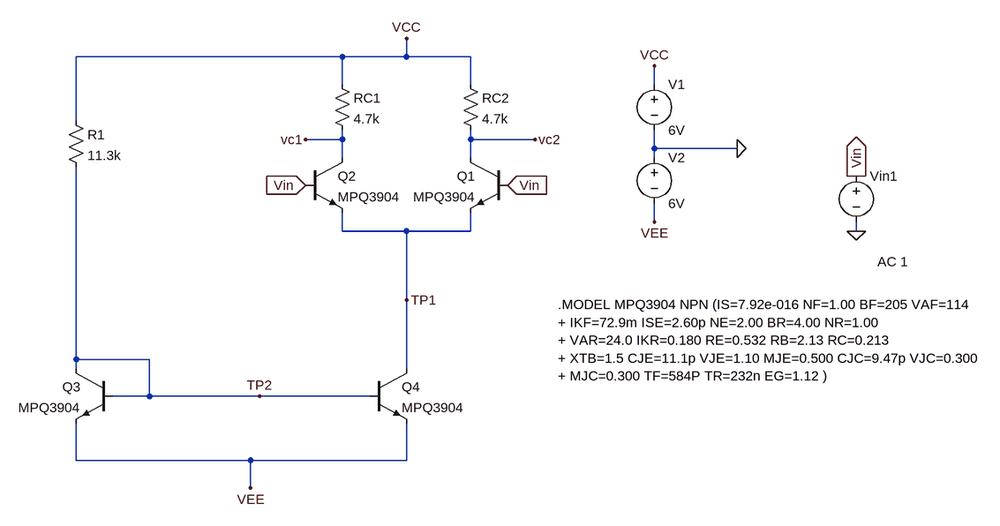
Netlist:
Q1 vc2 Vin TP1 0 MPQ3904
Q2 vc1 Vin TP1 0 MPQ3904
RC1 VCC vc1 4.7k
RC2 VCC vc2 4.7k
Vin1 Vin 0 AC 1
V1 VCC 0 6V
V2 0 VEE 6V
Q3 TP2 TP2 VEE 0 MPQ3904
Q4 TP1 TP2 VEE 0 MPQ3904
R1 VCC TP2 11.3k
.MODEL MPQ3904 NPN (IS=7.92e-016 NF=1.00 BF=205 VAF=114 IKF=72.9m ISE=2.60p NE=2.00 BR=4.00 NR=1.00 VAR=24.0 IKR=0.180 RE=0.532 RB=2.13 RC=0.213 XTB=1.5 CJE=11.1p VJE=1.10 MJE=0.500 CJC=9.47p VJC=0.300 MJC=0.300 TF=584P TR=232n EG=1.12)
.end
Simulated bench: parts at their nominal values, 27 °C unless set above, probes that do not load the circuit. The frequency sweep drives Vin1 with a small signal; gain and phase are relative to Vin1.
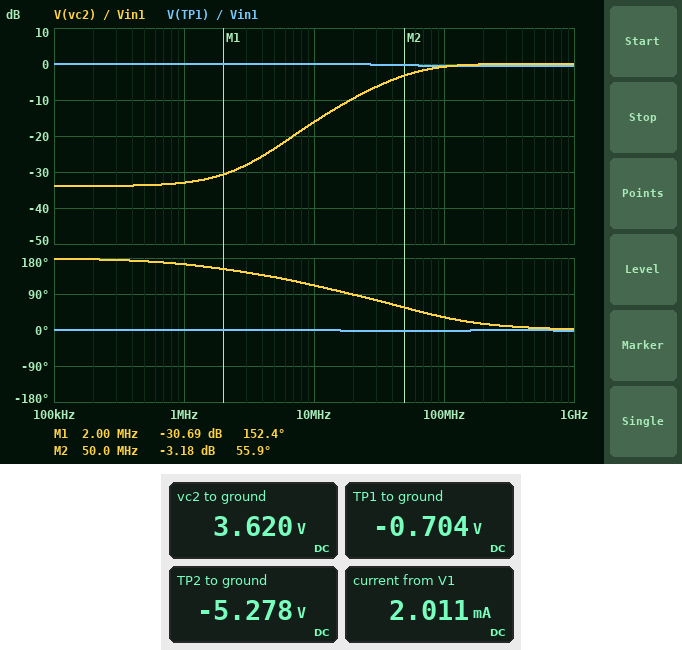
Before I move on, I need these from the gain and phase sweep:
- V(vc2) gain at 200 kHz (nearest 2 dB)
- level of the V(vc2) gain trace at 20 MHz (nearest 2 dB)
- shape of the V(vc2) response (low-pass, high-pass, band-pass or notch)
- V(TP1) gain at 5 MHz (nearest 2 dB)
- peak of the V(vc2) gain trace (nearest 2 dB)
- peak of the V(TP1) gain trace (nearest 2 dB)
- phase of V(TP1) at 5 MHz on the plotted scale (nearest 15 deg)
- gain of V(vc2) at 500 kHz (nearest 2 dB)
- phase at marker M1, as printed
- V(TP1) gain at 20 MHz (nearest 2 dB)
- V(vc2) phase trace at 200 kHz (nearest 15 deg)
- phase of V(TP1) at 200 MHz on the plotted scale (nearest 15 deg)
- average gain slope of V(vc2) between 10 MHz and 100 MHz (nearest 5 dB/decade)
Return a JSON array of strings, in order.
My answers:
["-34 dB", "-10 dB", "high-pass", "0 dB", "0 dB", "0 dB", "0 deg", "-34 dB", "152.4 deg", "0 dB", "180 deg", "0 deg", "15 dB/decade"]
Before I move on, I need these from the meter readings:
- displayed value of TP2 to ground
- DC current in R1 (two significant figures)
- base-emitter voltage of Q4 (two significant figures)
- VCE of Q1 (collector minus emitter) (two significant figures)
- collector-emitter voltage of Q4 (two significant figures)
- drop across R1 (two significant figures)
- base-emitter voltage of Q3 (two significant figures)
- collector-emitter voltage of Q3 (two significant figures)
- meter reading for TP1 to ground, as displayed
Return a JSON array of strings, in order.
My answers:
["-5.278 V", "1.0 mA", "720 mV", "4.3 V", "5.3 V", "11 V", "720 mV", "720 mV", "-0.704 V"]
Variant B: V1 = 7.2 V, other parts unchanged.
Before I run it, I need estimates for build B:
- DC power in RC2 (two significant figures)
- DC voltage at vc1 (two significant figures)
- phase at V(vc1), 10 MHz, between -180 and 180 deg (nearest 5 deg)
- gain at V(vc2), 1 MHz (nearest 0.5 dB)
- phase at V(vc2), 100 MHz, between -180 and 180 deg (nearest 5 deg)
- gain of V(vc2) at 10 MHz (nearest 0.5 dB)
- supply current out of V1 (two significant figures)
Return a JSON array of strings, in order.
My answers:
["1.5 mW", "4.6 V", "135 deg", "-32.0 dB", "35 deg", "-16.5 dB", "2.2 mA"]
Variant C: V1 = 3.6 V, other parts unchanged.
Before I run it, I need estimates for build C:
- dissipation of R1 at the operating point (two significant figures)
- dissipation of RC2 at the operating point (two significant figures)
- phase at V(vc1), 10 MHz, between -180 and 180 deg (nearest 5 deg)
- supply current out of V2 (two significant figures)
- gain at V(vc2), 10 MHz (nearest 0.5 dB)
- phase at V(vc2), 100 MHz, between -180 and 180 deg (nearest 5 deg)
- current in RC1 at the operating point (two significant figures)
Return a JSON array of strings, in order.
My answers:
["7.0 mW", "750 µW", "70 deg", "1.6 mA", "-12.0 dB", "25 deg", "400 µA"]
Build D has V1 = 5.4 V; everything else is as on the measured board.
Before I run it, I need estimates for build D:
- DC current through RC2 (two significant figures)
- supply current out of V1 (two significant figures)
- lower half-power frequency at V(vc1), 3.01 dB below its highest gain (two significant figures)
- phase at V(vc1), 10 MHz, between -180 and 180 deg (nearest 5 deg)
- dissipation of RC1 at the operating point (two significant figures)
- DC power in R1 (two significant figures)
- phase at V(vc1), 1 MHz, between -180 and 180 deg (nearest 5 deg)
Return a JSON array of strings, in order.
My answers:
["480 µA", "1.9 mA", "50 MHz", "100 deg", "1.1 mW", "10 mW", "150 deg"]
